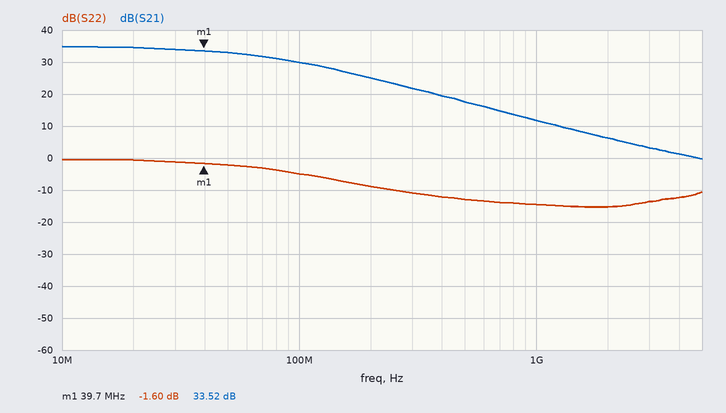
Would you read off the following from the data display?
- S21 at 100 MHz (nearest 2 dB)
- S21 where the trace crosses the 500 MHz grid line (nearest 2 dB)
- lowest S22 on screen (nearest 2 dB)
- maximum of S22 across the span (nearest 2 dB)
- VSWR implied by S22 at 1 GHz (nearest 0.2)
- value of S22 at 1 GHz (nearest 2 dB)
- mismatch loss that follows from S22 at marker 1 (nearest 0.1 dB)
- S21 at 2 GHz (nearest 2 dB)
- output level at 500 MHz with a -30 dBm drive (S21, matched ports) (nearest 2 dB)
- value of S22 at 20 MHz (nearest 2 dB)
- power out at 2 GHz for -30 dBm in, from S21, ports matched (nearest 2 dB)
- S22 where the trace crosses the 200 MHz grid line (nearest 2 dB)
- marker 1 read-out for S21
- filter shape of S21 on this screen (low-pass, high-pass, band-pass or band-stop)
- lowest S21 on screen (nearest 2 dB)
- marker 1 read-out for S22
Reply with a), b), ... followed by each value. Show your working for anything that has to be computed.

a) 30 dB
b) 18 dB
c) -16 dB
d) 0 dB
e) |Γ| = 10^(-14/20) = 0.1995; VSWR = (1 + 0.1995)/(1 − 0.1995) ≈ 1.50, so 1.4 to the nearest 0.2
f) -14 dB
g) −10 log10(1 − 10^(-1.6/10)) ≈ 5.1 dB
h) 6 dB
i) -30 dBm + (18 dB) = -12 dBm
j) 0 dB
k) -30 dBm + (6 dB) = -24 dBm
l) -8 dB
m) 33.52 dB
n) low-pass
o) 0 dB
p) -1.60 dB
